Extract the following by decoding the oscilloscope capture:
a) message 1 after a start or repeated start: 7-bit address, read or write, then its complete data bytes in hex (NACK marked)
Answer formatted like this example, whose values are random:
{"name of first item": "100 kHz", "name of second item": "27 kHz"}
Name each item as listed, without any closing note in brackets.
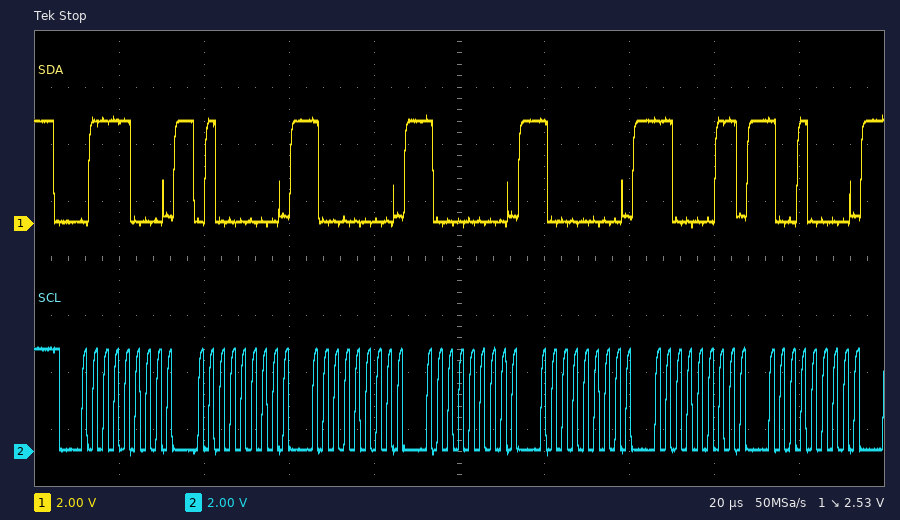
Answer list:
{"message 1 after a start or repeated start: 7-bit address, read or write, then its complete data bytes in hex": "0x3C write: 40 80 80 80 C3 90"}
